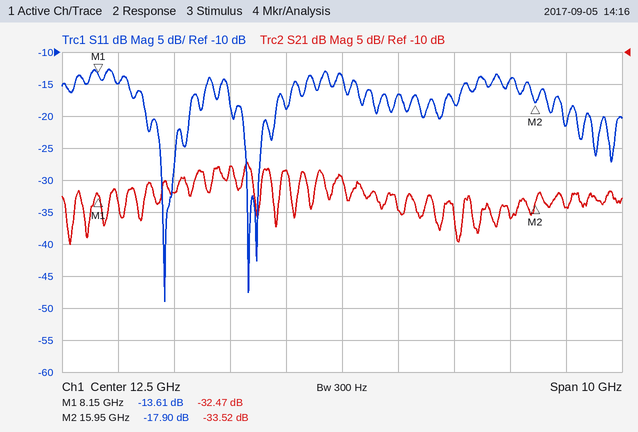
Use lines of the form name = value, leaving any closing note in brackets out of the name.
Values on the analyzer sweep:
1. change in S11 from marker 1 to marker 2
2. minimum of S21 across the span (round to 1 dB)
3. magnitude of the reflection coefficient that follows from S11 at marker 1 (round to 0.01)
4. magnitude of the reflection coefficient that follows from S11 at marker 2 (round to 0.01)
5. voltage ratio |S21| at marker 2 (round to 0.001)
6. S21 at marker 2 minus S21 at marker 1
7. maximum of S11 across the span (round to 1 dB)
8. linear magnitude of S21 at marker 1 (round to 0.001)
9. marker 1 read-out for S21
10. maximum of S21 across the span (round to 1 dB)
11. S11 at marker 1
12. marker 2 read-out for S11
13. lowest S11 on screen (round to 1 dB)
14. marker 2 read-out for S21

change in S11 from marker 1 to marker 2 = -4.29 dB
minimum of S21 across the span = -40 dB
magnitude of the reflection coefficient that follows from S11 at marker 1 = 0.21
magnitude of the reflection coefficient that follows from S11 at marker 2 = 0.13
voltage ratio |S21| at marker 2 = 0.021
S21 at marker 2 minus S21 at marker 1 = -1.05 dB
maximum of S11 across the span = -13 dB
linear magnitude of S21 at marker 1 = 0.024
marker 1 read-out for S21 = -32.47 dB
maximum of S21 across the span = -27 dB
S11 at marker 1 = -13.61 dB
marker 2 read-out for S11 = -17.90 dB
lowest S11 on screen = -49 dB
marker 2 read-out for S21 = -33.52 dB
